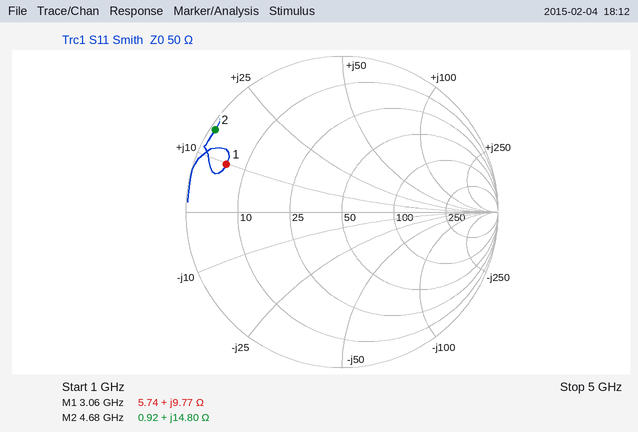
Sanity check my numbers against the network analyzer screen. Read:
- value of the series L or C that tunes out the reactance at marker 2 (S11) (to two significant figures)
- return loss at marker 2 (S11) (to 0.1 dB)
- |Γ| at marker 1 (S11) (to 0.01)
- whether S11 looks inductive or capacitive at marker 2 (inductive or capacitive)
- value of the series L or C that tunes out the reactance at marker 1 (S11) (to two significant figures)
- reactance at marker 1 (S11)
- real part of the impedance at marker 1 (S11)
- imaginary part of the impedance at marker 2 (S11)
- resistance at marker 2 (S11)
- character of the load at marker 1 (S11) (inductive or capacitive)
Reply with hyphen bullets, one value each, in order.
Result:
- 2.3 pF
- 0.3 dB
- 0.80
- inductive
- 5.3 pF
- +9.77 Ω
- 5.74 Ω
- +14.80 Ω
- 0.92 Ω
- inductive
